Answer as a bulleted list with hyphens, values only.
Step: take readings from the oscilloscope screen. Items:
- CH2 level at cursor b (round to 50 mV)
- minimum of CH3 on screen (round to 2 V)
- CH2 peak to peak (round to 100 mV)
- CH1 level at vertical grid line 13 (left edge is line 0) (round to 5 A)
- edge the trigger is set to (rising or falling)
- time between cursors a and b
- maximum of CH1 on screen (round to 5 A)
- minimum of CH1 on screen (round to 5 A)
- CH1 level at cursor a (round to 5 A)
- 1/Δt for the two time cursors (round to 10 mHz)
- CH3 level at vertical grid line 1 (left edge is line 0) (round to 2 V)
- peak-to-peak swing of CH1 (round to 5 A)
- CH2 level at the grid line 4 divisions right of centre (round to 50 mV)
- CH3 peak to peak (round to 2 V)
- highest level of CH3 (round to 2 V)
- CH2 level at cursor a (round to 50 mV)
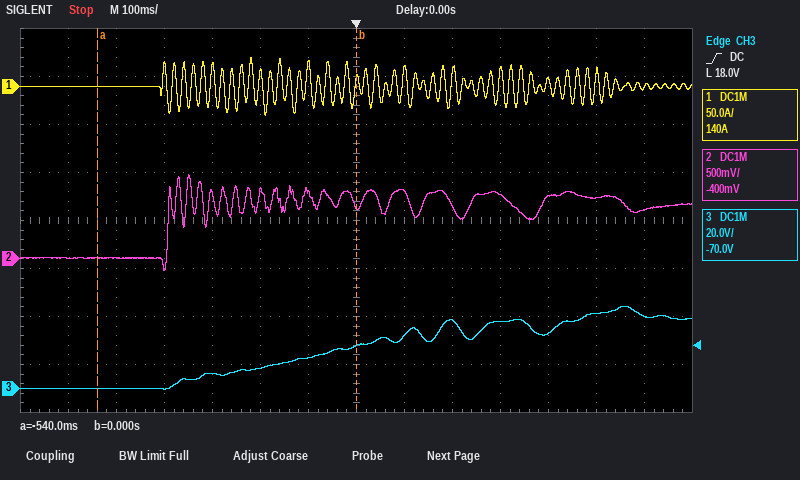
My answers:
- 550 mV
- 0 V
- 1.00 V
- 0 A
- rising
- 540 ms
- 30 A
- -30 A
- 0 A
- 1.85 Hz
- 0 V
- 60 A
- 650 mV
- 34 V
- 34 V
- 0 mV
